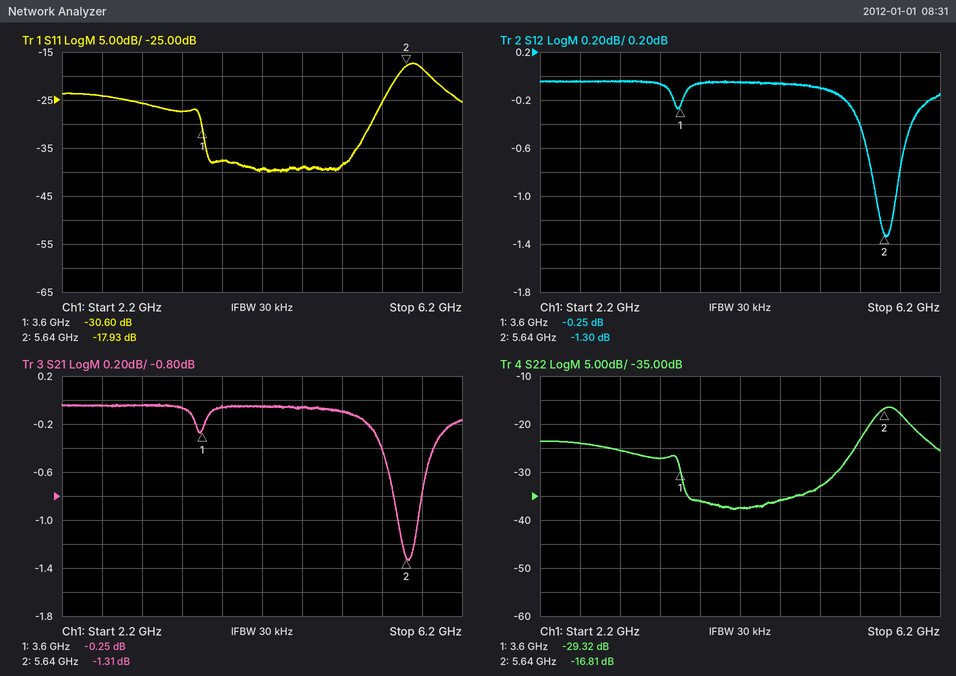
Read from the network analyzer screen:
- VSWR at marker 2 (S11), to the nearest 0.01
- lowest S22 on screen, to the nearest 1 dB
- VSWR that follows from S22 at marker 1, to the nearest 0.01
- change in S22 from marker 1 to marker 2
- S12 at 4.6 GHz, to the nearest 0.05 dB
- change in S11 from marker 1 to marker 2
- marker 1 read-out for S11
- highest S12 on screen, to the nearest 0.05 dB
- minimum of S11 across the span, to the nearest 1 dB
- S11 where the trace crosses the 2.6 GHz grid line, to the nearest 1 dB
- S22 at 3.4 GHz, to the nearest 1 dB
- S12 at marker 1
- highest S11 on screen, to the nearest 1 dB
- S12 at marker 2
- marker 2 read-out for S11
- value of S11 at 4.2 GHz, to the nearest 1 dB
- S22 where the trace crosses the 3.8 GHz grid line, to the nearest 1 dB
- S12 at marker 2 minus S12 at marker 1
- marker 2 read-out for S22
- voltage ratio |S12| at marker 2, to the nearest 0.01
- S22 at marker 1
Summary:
1.29
-38 dB
1.07
12.51 dB
-0.05 dB
12.67 dB
-30.60 dB
-0.05 dB
-40 dB
-24 dB
-27 dB
-0.25 dB
-17 dB
-1.30 dB
-17.93 dB
-39 dB
-36 dB
-1.05 dB
-16.81 dB
0.86
-29.32 dB
